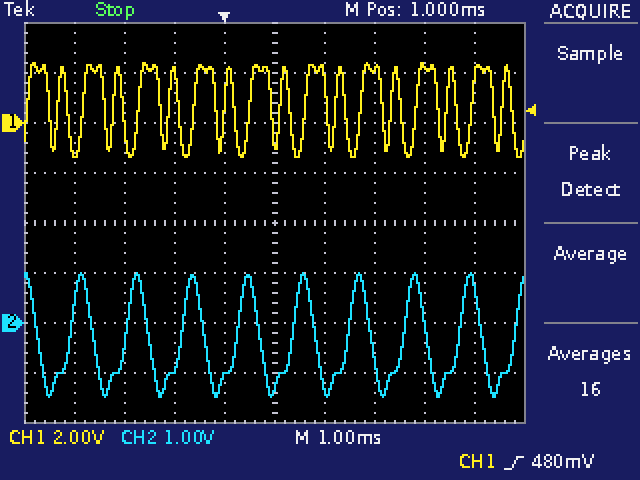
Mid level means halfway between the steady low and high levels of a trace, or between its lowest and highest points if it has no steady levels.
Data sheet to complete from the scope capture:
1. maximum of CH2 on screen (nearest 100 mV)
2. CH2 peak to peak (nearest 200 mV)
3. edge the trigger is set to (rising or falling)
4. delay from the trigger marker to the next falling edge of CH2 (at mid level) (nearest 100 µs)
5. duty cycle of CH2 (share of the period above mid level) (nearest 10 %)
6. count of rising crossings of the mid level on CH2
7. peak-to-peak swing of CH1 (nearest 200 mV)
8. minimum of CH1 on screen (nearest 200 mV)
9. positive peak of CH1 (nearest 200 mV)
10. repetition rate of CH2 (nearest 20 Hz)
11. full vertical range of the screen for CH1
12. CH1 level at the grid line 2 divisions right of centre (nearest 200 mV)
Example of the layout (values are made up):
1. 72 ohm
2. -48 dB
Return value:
1. 1.0 V
2. 2.4 V
3. rising
4. 700 µs
5. 40 %
6. 9
7. 3.8 V
8. -1.4 V
9. 2.4 V
10. 900 Hz
11. 16 V
12. 2.2 V
